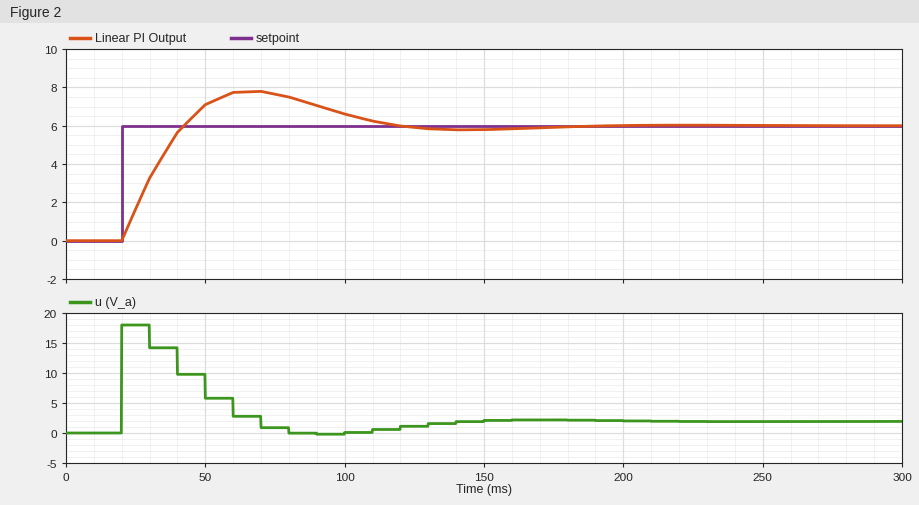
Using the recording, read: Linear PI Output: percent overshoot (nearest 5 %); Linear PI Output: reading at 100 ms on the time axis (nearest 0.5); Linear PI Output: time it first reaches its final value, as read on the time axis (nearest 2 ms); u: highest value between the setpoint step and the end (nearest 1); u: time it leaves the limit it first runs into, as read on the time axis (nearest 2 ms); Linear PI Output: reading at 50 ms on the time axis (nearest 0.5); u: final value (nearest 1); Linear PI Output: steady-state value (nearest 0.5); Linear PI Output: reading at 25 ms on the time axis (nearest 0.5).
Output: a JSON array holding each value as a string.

["30 %", "6.5", "42 ms", "18", "30 ms", "7.0", "2", "6.0", "1.5"]
